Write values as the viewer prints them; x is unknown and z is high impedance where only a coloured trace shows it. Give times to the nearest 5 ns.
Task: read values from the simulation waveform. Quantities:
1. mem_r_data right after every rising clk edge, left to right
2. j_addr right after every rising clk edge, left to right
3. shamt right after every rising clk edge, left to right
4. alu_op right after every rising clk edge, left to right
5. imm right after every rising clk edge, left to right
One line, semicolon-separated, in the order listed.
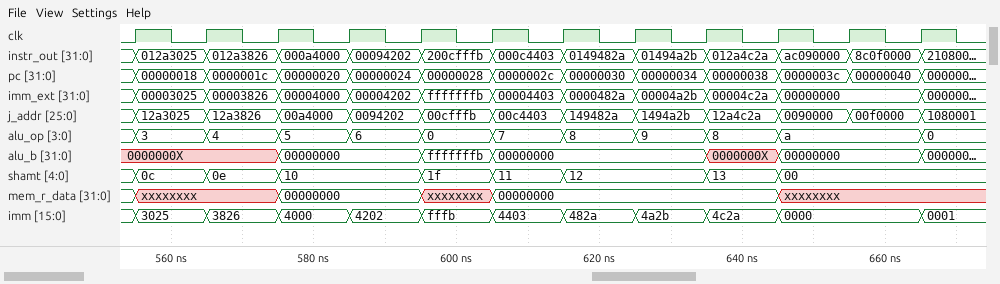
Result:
xxxxxxxx, xxxxxxxx, 00000000, 00000000, xxxxxxxx, 00000000, 00000000, 00000000, 00000000, xxxxxxxx, xxxxxxxx, xxxxxxxx; 12a3025, 12a3826, 00a4000, 0094202, 00cfffb, 00c4403, 149482a, 1494a2b, 12a4c2a, 0090000, 00f0000, 1080001; 0c, 0e, 10, 10, 1f, 11, 12, 12, 13, 00, 00, 00; 3, 4, 5, 6, 0, 7, 8, 9, 8, a, a, 0; 3025, 3826, 4000, 4202, fffb, 4403, 482a, 4a2b, 4c2a, 0000, 0000, 0001
